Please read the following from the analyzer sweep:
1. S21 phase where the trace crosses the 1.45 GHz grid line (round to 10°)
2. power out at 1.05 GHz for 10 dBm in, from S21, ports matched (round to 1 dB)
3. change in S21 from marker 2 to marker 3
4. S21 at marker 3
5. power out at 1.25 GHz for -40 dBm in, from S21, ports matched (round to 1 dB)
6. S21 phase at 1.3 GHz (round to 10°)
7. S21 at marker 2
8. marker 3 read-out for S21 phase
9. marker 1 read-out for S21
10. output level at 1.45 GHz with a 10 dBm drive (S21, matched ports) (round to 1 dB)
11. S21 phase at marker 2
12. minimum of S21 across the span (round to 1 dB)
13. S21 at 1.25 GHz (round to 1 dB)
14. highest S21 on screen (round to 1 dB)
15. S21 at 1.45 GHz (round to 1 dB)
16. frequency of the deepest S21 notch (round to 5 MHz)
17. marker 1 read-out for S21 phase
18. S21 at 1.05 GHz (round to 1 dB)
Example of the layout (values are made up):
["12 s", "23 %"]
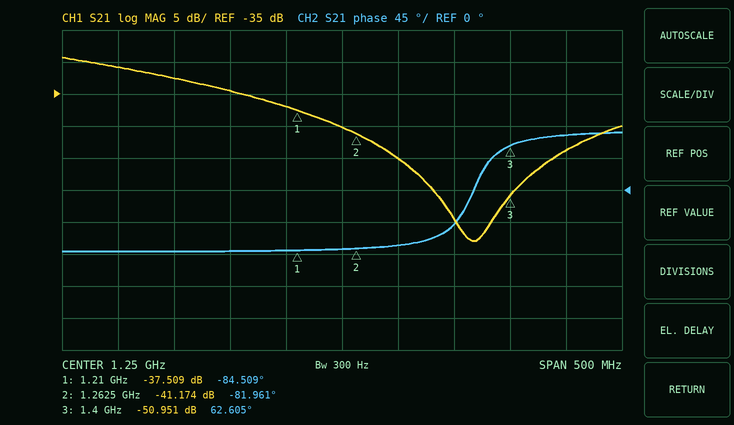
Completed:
["80°", "-21 dBm", "-9.777 dB", "-50.951 dB", "-80 dBm", "-80°", "-41.174 dB", "62.605°", "-37.509 dB", "-34 dBm", "-81.961°", "-58 dB", "-40 dB", "-29 dB", "-44 dB", "1.365 GHz", "-84.509°", "-31 dB"]
